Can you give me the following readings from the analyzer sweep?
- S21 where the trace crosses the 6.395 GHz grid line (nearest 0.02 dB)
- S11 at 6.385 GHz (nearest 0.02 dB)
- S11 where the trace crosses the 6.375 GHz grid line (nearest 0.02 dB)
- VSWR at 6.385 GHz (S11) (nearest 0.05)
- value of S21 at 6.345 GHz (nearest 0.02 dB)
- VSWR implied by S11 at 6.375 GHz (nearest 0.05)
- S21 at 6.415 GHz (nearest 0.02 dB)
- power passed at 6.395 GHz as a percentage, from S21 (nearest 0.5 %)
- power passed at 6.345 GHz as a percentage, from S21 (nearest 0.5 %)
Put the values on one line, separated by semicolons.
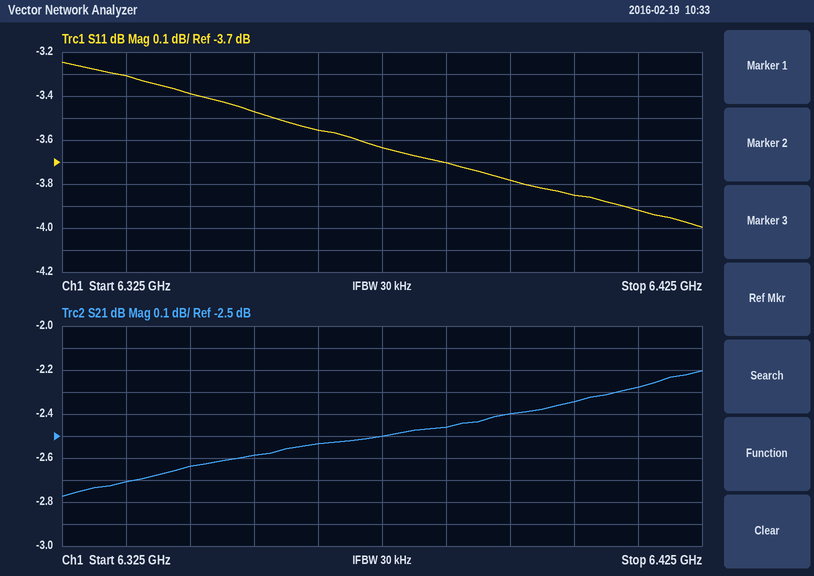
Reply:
-2.40 dB; -3.70 dB; -3.64 dB; 4.75; -2.64 dB; 4.85; -2.28 dB; 57.5 %; 54.5 %
